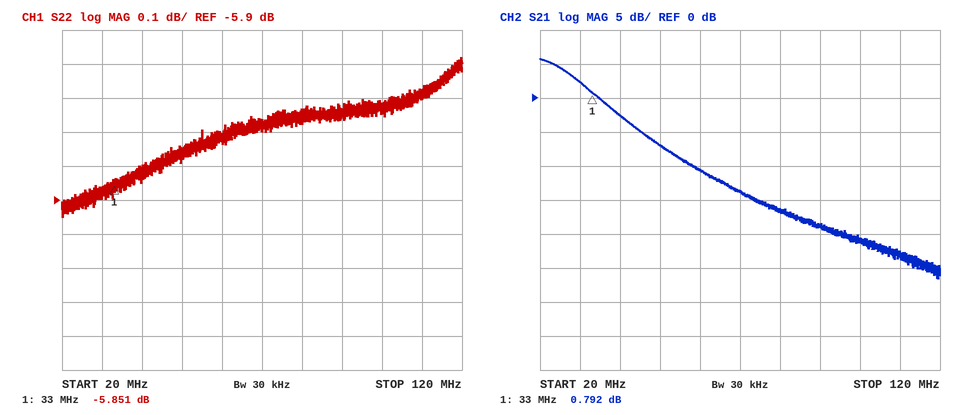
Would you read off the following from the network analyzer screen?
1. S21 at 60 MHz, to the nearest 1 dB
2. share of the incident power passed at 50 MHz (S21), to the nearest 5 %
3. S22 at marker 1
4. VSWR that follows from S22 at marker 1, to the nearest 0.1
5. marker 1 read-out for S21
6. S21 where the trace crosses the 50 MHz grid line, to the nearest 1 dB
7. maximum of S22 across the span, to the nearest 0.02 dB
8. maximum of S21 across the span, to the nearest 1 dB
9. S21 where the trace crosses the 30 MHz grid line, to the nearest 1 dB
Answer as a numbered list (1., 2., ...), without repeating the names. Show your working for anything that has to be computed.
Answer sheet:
1. -11 dB
2. 10^(-7/10) ≈ 20 %
3. -5.851 dB
4. (1 + 0.5099)/(1 − 0.5099) ≈ 3.1
5. 0.792 dB
6. -7 dB
7. -5.48 dB
8. 6 dB
9. 2 dB
